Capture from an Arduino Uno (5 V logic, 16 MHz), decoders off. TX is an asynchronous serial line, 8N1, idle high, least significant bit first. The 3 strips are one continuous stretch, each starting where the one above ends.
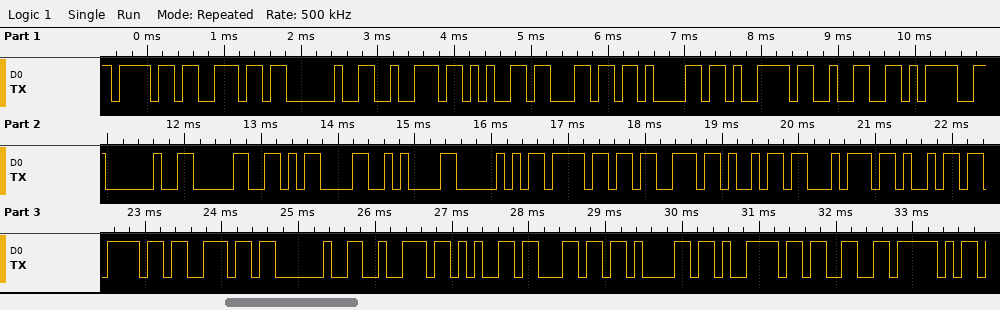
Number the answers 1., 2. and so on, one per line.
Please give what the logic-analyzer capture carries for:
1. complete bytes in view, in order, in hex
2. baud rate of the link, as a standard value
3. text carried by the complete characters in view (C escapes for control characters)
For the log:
1. 6F 6E 20 72 65 6C 61 79 32 3D 20 30 0D 0A 50 6F 73 69 74 69 6F 6E 20 72 65 6C 61 79 33 5F
2. 9600 baud
3. "on relay2= 0\r\nPosition relay3_"
